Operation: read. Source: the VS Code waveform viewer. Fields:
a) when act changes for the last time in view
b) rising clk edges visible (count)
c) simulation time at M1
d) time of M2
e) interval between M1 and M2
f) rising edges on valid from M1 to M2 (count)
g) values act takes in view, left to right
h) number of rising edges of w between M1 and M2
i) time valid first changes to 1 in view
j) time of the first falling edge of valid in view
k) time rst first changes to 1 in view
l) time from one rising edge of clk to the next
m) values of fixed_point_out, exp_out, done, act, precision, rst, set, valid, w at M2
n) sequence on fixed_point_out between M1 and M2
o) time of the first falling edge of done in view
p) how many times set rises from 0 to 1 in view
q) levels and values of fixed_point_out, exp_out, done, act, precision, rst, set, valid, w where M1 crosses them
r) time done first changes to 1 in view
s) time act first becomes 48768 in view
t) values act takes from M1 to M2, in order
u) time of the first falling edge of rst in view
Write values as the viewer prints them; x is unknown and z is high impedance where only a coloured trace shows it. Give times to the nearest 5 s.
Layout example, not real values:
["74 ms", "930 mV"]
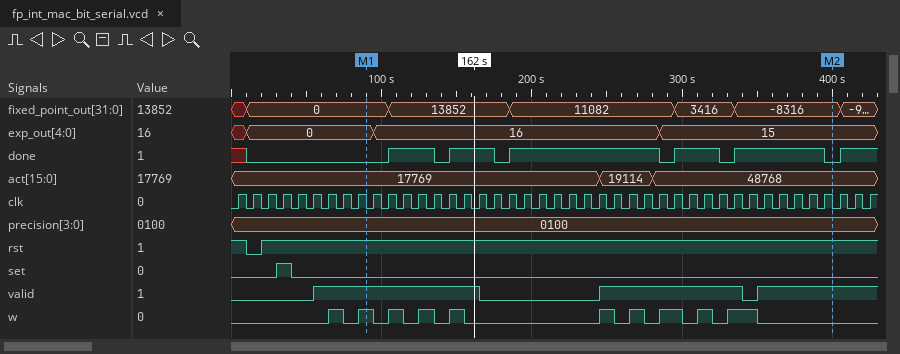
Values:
["280 s", "43", "90 s", "400 s", "310 s", "2", "17769, 19114, 48768", "8", "55 s", "165 s", "20 s", "10 s", "fixed_point_out=-8316, exp_out=15, done=0, act=48768, precision=0100, rst=1, set=0, valid=1, w=0", "0, 13852, 11082, 3416, -8316", "135 s", "1", "fixed_point_out=0, exp_out=0, done=0, act=17769, precision=0100, rst=1, set=0, valid=1, w=1", "105 s", "280 s", "17769, 19114, 48768", "10 s"]
